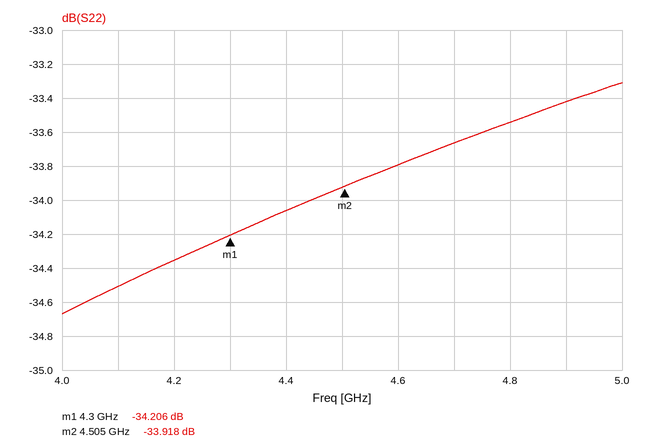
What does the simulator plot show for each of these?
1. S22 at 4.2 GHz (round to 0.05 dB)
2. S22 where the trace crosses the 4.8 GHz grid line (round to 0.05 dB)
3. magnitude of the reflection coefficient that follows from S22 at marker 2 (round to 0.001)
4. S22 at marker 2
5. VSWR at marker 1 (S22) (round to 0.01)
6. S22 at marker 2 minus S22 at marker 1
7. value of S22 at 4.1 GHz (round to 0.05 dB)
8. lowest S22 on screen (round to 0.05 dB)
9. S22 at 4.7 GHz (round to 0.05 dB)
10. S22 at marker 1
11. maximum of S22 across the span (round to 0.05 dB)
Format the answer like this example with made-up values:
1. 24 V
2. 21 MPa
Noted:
1. -34.35 dB
2. -33.55 dB
3. 0.020
4. -33.918 dB
5. 1.04
6. 0.288 dB
7. -34.50 dB
8. -34.65 dB
9. -33.65 dB
10. -34.206 dB
11. -33.30 dB
